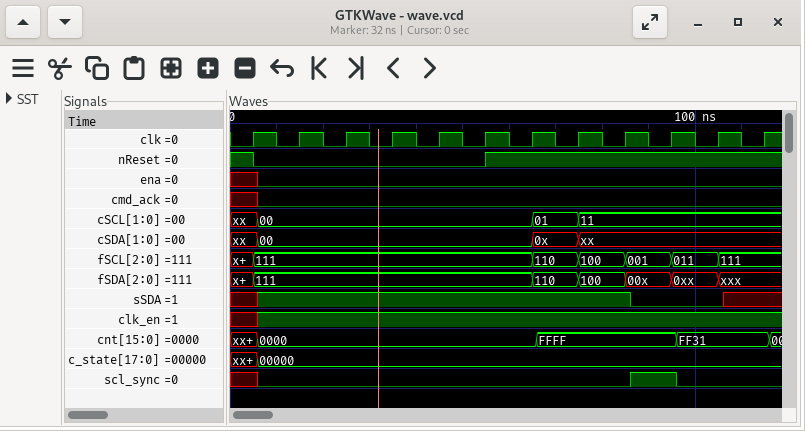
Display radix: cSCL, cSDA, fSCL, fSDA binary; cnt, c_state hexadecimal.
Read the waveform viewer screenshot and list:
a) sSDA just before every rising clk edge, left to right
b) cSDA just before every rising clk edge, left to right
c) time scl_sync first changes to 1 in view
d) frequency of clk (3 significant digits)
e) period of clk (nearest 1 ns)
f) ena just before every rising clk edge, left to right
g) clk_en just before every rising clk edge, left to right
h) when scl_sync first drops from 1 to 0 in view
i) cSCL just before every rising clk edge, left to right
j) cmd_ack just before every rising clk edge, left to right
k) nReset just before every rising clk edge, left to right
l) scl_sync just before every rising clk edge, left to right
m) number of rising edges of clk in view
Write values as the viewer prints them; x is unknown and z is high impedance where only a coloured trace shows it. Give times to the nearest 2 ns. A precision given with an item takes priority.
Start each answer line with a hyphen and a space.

- x 1 1 1 1 1 1 1 1 0 0 x
- xx, 00, 00, 00, 00, 00, 00, 0x, xx, xx, xx, xx
- 86 ns
- 100 MHz
- 10 ns
- x 0 0 0 0 0 0 0 0 0 0 0
- x 1 1 1 1 1 1 1 1 1 1 1
- 96 ns
- xx, 00, 00, 00, 00, 00, 00, 01, 11, 11, 11, 11
- x 0 0 0 0 0 0 0 0 0 0 0
- 1 0 0 0 0 0 1 1 1 1 1 1
- x 0 0 0 0 0 0 0 0 1 0 0
- 12
